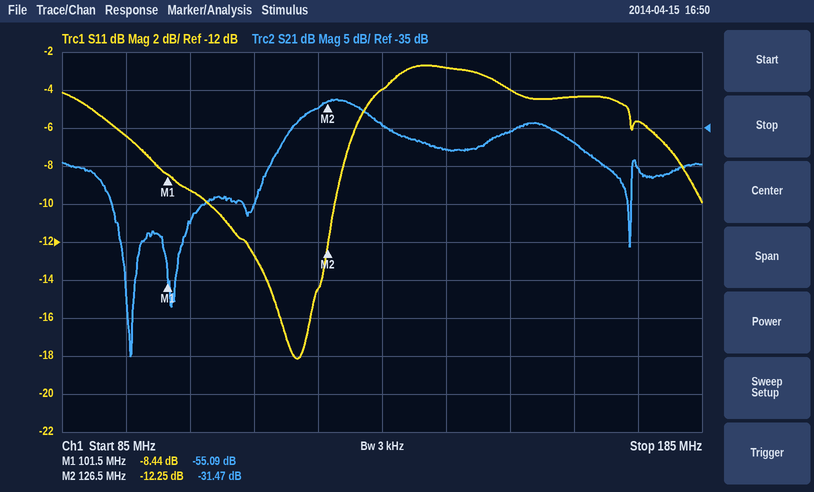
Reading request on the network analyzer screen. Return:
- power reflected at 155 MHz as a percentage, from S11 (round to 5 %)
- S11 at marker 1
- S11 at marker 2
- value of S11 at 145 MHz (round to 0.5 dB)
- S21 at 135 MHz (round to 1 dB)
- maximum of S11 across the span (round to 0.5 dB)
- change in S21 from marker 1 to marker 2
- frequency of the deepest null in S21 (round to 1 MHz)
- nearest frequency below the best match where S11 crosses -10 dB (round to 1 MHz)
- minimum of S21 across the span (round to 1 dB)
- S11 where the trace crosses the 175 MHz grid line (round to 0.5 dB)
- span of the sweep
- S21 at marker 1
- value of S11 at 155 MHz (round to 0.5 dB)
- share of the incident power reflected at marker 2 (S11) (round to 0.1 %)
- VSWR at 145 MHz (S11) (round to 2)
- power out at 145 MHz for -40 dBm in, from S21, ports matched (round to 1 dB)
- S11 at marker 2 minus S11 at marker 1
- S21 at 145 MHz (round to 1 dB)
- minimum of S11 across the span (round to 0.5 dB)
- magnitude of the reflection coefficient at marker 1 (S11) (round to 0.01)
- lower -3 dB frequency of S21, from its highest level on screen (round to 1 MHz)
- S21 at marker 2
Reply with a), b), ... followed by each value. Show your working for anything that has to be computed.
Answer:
a) 10^(-4/10) ≈ 40 %
b) -8.44 dB
c) -12.25 dB
d) -3.0 dB
e) -35 dB
f) -2.5 dB
g) -31.47 − (-55.09) = 23.62 dB
h) 96 MHz
i) 108 MHz
j) -65 dB
k) -5.5 dB
l) 100 MHz
m) -55.09 dB
n) -4.0 dB
o) 10^(-12.25/10) ≈ 6.0 %
p) |Γ| = 10^(-3/20) = 0.7079; VSWR = (1 + 0.7079)/(1 − 0.7079) ≈ 6
q) -40 dBm + (-38 dB) = -78 dBm
r) -12.25 − (-8.44) = -3.81 dB
s) -38 dB
t) -18.0 dB
u) 10^(-8.44/20) ≈ 0.38
v) 122 MHz
w) -31.47 dB
